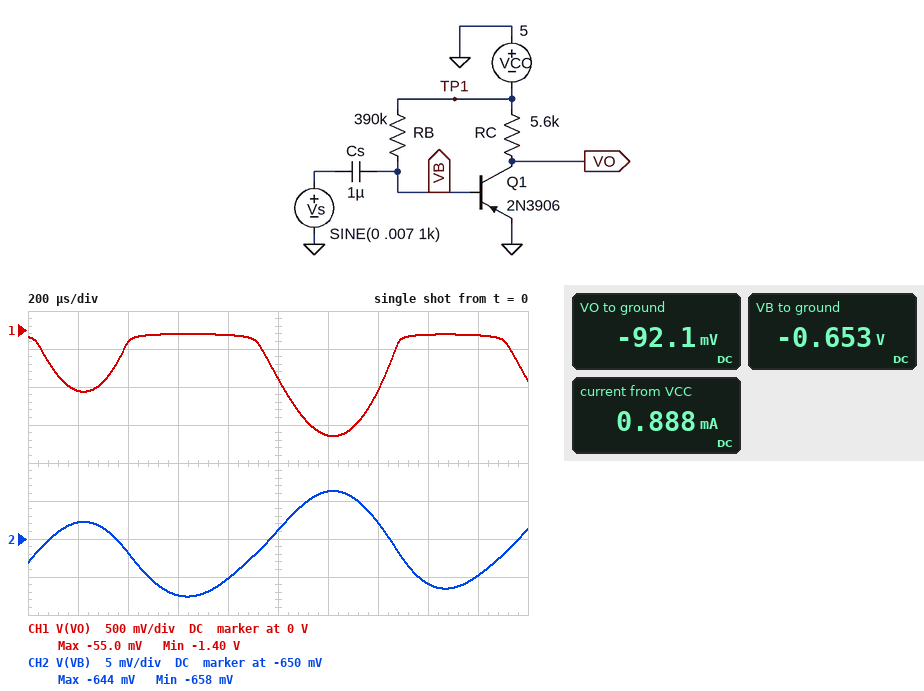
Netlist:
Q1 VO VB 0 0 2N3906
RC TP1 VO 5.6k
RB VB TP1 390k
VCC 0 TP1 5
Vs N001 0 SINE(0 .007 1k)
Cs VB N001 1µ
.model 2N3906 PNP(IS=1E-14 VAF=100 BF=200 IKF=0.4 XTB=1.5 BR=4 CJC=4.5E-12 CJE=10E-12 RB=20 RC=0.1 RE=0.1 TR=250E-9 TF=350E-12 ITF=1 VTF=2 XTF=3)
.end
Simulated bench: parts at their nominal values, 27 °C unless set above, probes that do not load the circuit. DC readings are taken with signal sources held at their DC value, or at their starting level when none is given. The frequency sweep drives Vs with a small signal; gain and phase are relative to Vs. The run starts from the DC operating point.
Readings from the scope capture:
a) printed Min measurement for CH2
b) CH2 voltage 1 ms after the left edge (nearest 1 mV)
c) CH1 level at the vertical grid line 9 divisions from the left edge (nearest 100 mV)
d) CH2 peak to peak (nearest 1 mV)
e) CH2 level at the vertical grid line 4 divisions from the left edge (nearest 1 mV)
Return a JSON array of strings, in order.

["-658 mV", "-649 mV", "-100 mV", "14 mV", "-655 mV"]
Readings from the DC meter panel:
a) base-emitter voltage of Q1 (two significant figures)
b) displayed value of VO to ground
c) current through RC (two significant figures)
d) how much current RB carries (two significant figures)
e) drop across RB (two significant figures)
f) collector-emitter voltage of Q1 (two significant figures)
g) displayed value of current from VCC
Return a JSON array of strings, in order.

["-650 mV", "-92.1 mV", "880 µA", "11 µA", "4.3 V", "-92 mV", "0.888 mA"]
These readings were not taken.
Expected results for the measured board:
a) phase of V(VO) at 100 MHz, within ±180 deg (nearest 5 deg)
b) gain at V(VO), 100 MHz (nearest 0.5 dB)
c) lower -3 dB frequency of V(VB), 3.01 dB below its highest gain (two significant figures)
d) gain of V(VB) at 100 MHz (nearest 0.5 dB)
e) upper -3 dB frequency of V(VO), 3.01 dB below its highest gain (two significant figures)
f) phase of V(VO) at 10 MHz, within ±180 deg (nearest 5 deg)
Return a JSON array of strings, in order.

["0 deg", "-4.5 dB", "900 Hz", "0 dB", "590 kHz", "65 deg"]
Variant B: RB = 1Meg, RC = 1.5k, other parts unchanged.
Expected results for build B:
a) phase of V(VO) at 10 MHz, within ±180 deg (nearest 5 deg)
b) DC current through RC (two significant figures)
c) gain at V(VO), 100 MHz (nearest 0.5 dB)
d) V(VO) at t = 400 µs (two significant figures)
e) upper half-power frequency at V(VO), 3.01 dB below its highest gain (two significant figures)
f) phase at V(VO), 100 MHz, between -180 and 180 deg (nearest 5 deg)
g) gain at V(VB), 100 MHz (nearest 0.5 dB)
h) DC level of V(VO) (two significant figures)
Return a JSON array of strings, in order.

["155 deg", "890 µA", "21.0 dB", "-3.8 V", "23 MHz", "90 deg", "0 dB", "-3.7 V"]
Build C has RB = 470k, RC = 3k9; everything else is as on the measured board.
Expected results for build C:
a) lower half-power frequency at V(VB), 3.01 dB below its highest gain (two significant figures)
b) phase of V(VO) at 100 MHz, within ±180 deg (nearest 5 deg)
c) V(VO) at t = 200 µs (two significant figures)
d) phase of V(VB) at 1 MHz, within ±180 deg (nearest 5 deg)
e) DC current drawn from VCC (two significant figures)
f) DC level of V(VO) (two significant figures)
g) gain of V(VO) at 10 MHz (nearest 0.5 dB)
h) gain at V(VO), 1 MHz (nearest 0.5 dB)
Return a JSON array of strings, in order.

["960 Hz", "20 deg", "-1.0 V", "0 deg", "1.3 mA", "-120 mV", "10.5 dB", "29.0 dB"]
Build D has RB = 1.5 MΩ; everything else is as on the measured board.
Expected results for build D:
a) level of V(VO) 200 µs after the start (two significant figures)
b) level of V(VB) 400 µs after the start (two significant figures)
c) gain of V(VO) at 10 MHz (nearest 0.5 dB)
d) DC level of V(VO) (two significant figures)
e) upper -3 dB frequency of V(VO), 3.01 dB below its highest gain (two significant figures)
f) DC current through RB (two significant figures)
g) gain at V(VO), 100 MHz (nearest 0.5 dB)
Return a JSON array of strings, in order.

["-2.4 V", "-640 mV", "36.0 dB", "-1.7 V", "6.0 MHz", "2.9 µA", "17.0 dB"]
